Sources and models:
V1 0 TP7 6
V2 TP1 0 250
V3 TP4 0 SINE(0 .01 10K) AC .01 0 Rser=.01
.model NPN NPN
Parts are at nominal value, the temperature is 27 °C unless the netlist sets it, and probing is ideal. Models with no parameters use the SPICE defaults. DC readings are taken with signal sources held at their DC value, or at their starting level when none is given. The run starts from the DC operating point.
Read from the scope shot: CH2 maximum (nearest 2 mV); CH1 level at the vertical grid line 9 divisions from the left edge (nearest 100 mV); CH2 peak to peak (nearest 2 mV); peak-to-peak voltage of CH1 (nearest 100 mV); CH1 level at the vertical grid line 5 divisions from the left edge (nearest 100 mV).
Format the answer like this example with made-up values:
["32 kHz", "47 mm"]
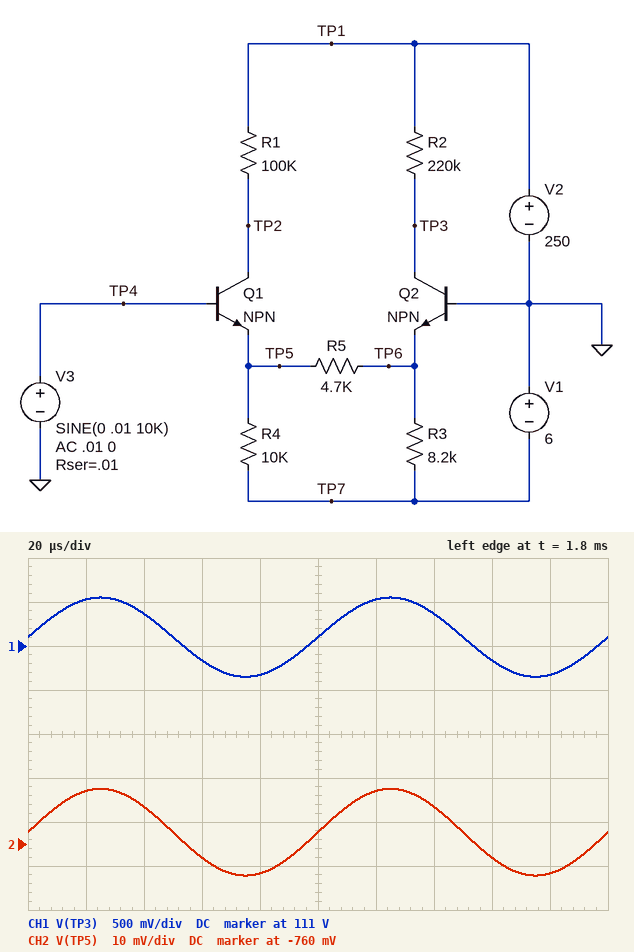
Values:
["-748 mV", "110.7 V", "20 mV", "900 mV", "111.1 V"]
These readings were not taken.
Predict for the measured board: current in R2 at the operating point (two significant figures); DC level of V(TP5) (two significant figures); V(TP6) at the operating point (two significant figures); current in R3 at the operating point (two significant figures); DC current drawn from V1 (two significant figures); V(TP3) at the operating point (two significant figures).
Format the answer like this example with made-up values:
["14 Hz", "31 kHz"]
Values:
["630 µA", "-760 mV", "-760 mV", "640 µA", "1.2 mA", "110 V"]
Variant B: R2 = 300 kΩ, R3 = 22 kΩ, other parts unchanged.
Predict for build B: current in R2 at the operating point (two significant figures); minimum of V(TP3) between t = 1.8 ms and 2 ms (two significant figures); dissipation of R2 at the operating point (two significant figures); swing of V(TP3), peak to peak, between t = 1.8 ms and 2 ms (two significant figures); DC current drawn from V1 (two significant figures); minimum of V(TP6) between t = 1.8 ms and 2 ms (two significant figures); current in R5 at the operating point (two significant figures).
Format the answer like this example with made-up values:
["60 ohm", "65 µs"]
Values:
["240 µA", "180 V", "17 mW", "1.2 V", "760 µA", "-740 mV", "4.2 µA"]
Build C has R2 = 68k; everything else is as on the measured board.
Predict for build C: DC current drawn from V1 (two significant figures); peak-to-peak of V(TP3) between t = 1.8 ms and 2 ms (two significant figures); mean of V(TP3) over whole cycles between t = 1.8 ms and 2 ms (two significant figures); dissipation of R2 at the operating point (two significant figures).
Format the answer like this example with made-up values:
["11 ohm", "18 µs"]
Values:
["1.2 mA", "280 mV", "210 V", "27 mW"]
